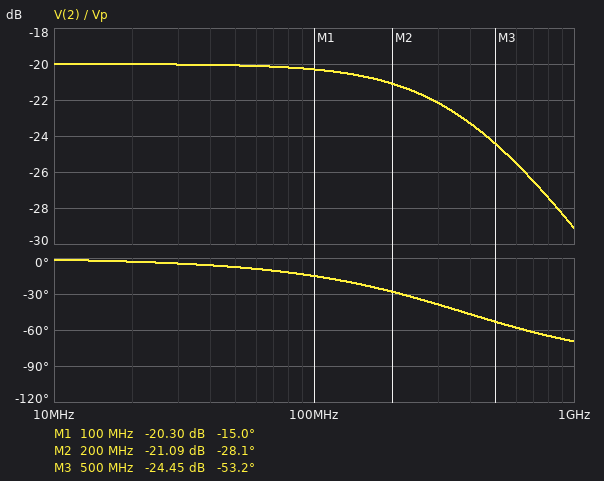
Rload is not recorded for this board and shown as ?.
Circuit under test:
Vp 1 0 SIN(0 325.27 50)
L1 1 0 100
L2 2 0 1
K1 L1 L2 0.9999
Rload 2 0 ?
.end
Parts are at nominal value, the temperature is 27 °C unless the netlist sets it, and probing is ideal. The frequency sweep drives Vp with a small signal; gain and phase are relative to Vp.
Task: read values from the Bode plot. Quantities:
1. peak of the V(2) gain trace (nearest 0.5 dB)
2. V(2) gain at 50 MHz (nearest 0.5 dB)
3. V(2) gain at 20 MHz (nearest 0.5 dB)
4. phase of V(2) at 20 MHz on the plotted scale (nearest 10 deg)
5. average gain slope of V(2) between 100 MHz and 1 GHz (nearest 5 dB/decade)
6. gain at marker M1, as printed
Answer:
-20.0 dB
-20.0 dB
-20.0 dB
0 deg
-10 dB/decade
-20.30 dB
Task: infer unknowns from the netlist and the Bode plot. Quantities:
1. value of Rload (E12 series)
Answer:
470 kΩ
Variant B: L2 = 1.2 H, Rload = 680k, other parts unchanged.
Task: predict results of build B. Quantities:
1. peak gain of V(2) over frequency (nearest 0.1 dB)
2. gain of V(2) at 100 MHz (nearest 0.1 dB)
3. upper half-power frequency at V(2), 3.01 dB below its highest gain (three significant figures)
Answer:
-19.2 dB
-19.4 dB
451 MHz
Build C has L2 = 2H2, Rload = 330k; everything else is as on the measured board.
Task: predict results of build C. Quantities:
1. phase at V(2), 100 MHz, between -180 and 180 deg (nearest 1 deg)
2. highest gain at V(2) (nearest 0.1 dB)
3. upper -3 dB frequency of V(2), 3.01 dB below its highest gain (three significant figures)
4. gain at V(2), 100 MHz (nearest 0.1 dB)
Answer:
-40 deg
-16.6 dB
119 MHz
-18.9 dB
